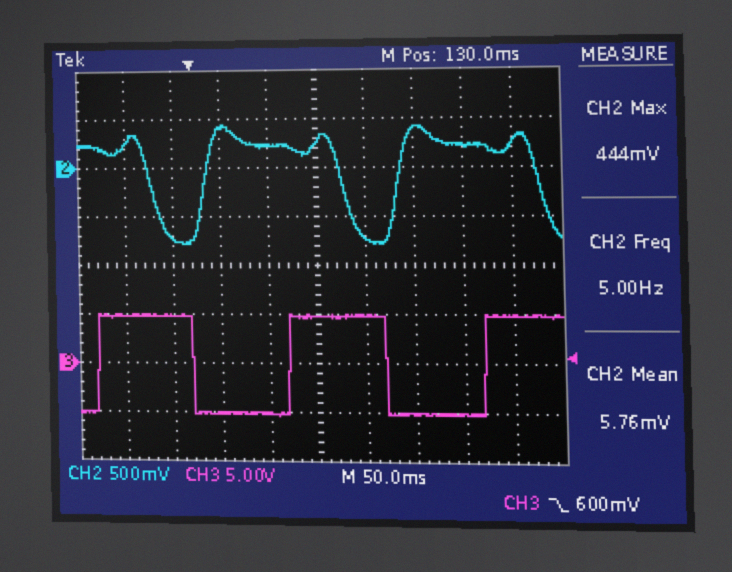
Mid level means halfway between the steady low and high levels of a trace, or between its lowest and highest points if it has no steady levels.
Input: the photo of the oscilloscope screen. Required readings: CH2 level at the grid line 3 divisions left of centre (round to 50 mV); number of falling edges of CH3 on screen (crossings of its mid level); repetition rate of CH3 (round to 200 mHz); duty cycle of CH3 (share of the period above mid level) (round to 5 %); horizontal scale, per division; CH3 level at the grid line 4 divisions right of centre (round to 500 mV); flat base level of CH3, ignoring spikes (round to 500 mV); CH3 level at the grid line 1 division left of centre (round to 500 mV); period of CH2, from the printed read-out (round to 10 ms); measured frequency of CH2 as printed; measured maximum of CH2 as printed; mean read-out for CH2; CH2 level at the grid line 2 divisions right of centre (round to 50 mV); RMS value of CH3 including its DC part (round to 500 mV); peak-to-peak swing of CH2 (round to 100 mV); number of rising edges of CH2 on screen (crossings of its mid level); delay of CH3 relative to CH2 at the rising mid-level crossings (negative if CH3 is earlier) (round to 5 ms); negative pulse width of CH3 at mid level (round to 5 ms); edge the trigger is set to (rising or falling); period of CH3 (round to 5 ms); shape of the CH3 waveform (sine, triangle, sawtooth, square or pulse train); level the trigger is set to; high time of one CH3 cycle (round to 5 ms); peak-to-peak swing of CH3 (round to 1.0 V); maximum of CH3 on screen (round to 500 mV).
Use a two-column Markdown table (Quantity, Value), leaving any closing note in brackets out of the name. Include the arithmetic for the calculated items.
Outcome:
| Quantity | Value |
|---|---|
| CH2 level at the grid line 3 divisions left of centre | -700 mV |
| number of falling edges of CH3 on screen | 2 |
| repetition rate of CH3 | 1 / 200 ms ≈ 5.0 Hz |
| duty cycle of CH3 (share of the period above mid level) | 100 ms / 200 ms ≈ 50 % |
| horizontal scale, per division | 50 ms |
| CH3 level at the grid line 4 divisions right of centre | 5.0 V |
| flat base level of CH3, ignoring spikes | -5.0 V |
| CH3 level at the grid line 1 division left of centre | -5.0 V |
| period of CH2, from the printed read-out | 1 / 5.00 Hz ≈ 200 ms |
| measured frequency of CH2 as printed | 5.00 Hz |
| measured maximum of CH2 as printed | 444 mV |
| mean read-out for CH2 | 5.76 mV |
| CH2 level at the grid line 2 divisions right of centre | 400 mV |
| RMS value of CH3 including its DC part | √(0.5 × (5.0 V)² + 0.5 × (-5.0 V)²) ≈ 5.0 V |
| peak-to-peak swing of CH2 | 1.20 V |
| number of rising edges of CH2 on screen | 2 |
| delay of CH3 relative to CH2 at the rising mid-level crossings (negative if CH3 is earlier) | +85 ms |
| negative pulse width of CH3 at mid level | 100 ms |
| edge the trigger is set to | falling |
| period of CH3 | 200 ms |
| shape of the CH3 waveform | square |
| level the trigger is set to | 600 mV |
| high time of one CH3 cycle | 100 ms |
| peak-to-peak swing of CH3 | 10.0 V |
| maximum of CH3 on screen | 5.0 V |
